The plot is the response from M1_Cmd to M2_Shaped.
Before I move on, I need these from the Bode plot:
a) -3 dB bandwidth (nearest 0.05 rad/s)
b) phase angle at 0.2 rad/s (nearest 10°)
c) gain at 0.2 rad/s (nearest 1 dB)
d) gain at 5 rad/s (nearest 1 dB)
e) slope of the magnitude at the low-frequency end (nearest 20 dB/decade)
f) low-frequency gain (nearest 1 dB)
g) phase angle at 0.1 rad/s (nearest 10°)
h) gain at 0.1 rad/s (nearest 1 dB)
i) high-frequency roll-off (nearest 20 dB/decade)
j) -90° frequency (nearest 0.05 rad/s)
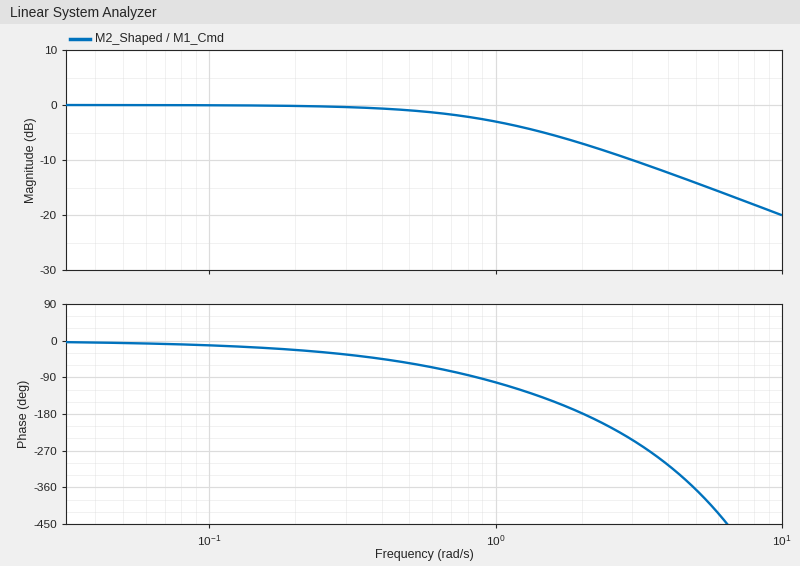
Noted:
1.00 rad/s
-20°
0 dB
-14 dB
0 dB/decade
0 dB
-10°
0 dB
-20 dB/decade
0.85 rad/s
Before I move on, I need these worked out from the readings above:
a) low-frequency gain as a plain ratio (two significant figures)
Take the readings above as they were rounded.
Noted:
1.0
